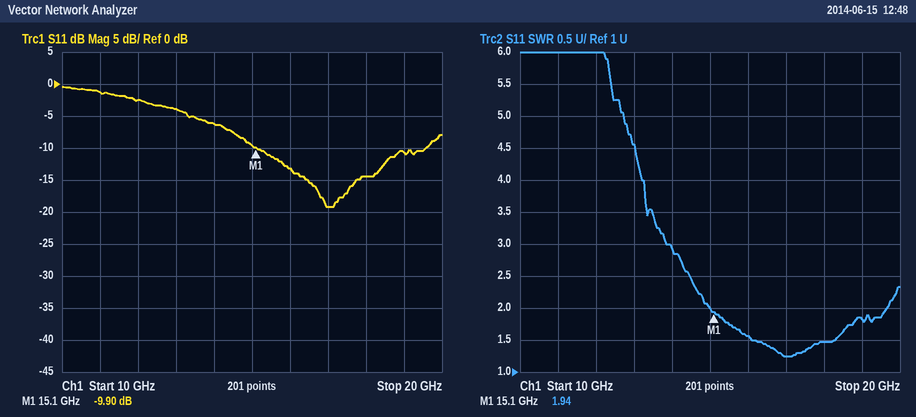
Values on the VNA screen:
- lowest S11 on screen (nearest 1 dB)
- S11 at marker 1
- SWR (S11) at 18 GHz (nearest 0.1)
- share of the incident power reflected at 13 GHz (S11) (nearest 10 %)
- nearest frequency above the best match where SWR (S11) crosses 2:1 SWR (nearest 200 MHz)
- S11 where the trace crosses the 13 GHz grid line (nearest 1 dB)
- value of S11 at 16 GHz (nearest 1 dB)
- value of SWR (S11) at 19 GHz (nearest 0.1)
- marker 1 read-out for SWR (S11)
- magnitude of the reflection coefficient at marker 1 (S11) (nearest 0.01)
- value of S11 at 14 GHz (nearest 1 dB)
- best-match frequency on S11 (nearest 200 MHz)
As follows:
-19 dB
-9.90 dB
1.5
40 %
19.6 GHz
-4 dB
-13 dB
1.8
1.94
0.32
-6 dB
17.0 GHz
